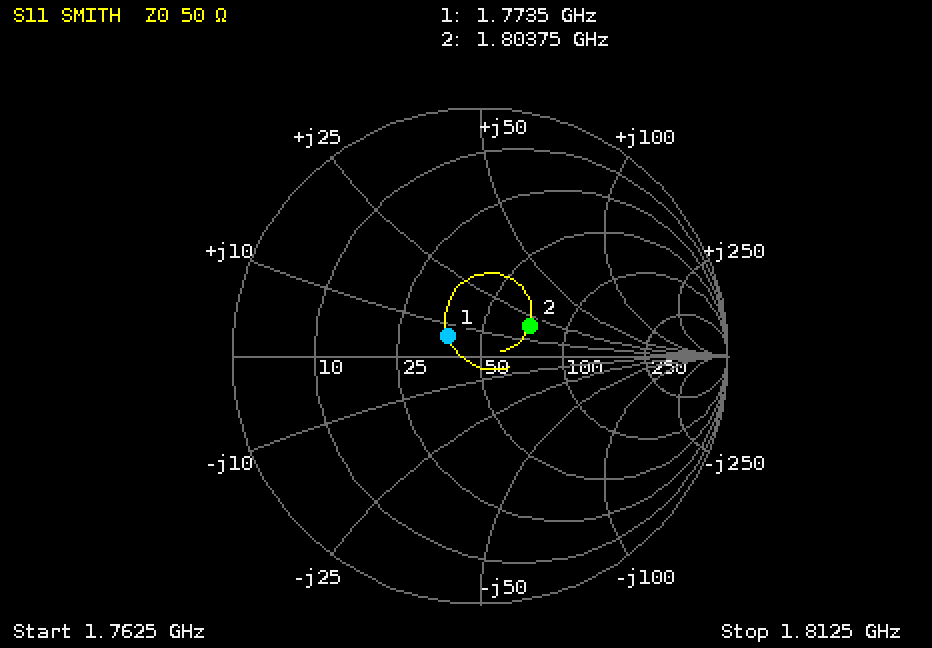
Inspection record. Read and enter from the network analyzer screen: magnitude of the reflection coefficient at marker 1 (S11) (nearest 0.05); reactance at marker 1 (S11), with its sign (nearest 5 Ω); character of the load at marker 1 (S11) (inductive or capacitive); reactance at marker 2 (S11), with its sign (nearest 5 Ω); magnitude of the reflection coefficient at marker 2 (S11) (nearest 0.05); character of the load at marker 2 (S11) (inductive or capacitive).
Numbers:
0.15
+5 Ω
inductive
+20 Ω
0.25
inductive
